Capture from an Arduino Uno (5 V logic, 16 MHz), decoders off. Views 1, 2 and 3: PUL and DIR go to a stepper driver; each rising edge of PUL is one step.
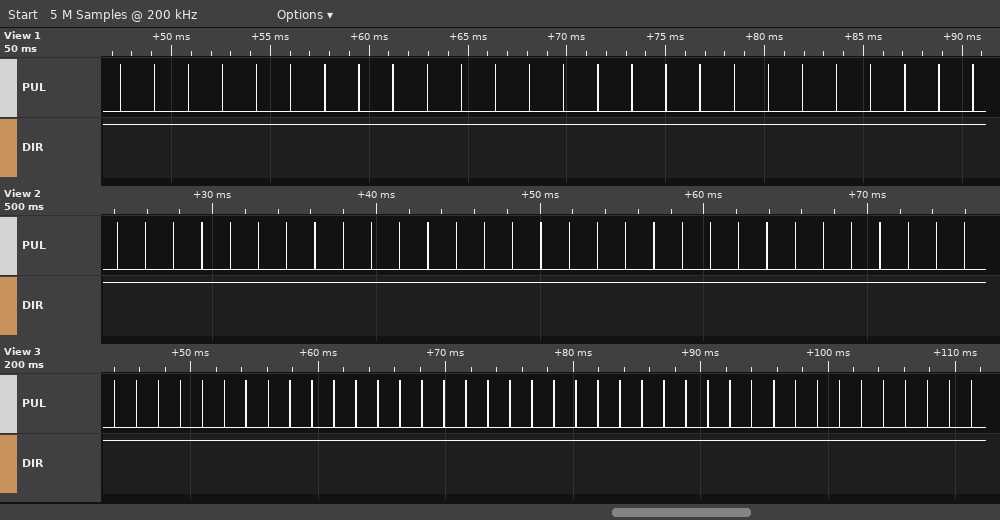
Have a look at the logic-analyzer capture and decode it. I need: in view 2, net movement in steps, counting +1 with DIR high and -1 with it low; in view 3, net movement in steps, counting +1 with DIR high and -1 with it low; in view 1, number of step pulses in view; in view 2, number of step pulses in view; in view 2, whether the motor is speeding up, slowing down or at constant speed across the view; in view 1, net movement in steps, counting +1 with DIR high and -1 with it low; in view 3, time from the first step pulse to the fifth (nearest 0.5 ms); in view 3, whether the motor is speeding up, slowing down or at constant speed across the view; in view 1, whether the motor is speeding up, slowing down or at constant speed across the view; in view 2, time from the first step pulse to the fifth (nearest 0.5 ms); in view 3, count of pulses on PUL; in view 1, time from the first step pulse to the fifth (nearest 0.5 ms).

+31
+40
26
31
constant speed
+26
7.0 ms
constant speed
constant speed
7.0 ms
40
7.0 ms
